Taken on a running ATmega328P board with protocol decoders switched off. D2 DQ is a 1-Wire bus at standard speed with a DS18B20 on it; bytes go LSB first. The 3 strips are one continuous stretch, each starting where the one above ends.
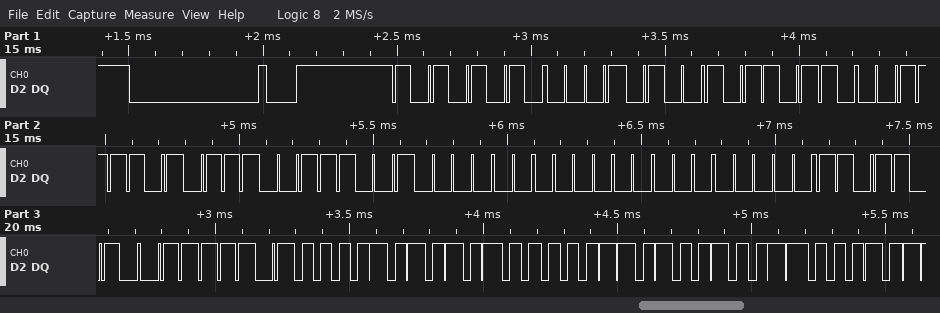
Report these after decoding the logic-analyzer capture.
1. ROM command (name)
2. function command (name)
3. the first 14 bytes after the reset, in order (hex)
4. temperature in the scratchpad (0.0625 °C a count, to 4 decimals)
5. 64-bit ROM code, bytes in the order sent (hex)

Match ROM
Read Scratchpad
55 28 6D BC CE 09 00 00 5B BE 50 05 4B 46
85.0000 °C
28 6D BC CE 09 00 00 5B
